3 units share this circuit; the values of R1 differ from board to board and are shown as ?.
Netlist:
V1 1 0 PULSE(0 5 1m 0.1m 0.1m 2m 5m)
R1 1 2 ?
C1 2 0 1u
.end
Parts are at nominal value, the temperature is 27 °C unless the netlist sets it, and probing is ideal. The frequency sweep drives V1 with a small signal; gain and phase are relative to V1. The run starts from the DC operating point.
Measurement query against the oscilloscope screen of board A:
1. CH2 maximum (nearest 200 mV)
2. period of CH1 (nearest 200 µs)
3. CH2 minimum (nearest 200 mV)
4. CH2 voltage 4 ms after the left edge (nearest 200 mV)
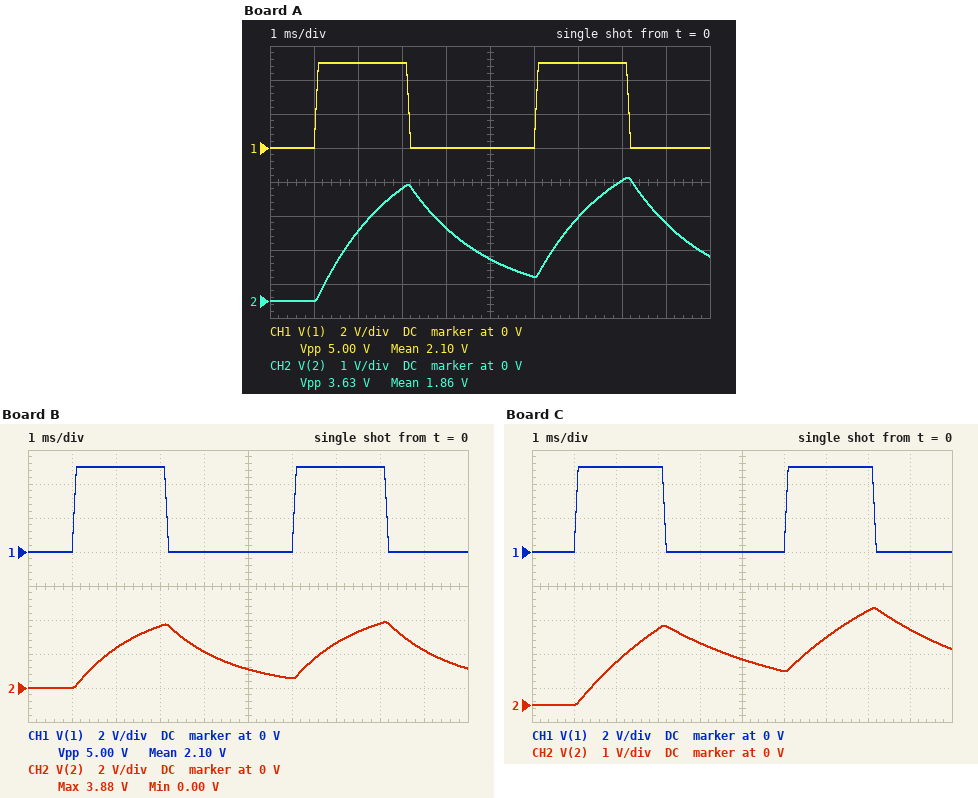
3.6 V
5.0 ms
0 V
2.2 V
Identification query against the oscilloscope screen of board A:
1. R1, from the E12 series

1.8 kΩ
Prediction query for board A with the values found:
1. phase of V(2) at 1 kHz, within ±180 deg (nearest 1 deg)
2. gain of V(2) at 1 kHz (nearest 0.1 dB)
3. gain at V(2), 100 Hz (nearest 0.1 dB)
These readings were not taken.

-85 deg
-21.1 dB
-3.6 dB
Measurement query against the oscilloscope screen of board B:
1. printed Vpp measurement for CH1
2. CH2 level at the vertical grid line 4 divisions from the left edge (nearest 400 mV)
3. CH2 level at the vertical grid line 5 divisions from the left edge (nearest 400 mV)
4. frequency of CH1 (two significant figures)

5.00 V
2.0 V
1.2 V
200 Hz
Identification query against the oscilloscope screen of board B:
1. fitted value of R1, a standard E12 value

1.5 kΩ
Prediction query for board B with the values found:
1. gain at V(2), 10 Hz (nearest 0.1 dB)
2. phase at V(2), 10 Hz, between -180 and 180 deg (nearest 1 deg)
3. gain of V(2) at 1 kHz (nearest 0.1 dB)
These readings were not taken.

0 dB
-5 deg
-19.5 dB
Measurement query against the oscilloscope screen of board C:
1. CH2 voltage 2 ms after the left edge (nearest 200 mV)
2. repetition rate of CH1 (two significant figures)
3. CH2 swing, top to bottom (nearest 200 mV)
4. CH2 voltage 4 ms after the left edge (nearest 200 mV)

1.2 V
200 Hz
2.8 V
1.8 V
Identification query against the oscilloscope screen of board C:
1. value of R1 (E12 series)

3.3 kΩ
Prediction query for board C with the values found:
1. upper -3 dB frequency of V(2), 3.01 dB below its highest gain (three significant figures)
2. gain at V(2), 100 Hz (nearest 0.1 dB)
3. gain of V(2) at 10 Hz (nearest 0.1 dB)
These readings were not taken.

48.2 Hz
-7.2 dB
-0.2 dB
